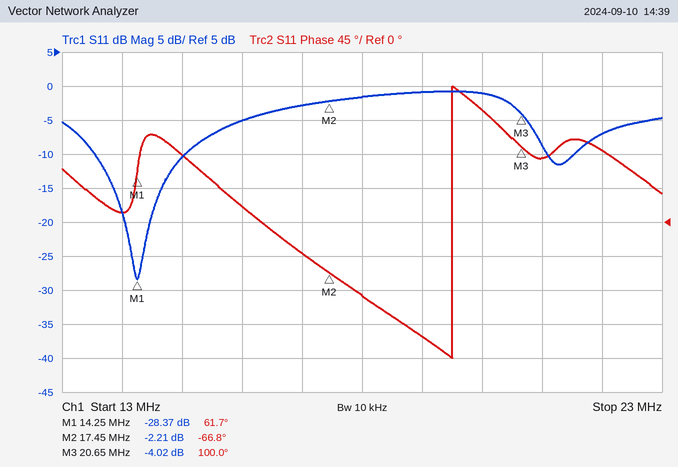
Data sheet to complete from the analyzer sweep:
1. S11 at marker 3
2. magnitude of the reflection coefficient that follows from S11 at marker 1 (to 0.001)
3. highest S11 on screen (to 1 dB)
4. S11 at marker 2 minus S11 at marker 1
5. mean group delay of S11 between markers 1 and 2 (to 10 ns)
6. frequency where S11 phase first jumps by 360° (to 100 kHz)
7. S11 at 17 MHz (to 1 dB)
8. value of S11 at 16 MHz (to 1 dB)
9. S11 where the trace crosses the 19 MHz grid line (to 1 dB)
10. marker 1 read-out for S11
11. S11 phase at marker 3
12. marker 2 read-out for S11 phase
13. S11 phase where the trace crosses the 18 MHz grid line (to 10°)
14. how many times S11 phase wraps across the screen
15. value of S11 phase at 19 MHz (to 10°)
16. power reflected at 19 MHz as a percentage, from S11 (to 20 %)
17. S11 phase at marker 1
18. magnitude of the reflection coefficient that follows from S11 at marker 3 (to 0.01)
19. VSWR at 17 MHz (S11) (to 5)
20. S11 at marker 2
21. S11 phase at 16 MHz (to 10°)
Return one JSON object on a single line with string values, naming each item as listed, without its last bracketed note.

{"S11 at marker 3": "-4.02 dB", "magnitude of the reflection coefficient that follows from S11 at marker 1": "0.038", "highest S11 on screen": "-1 dB", "S11 at marker 2 minus S11 at marker 1": "26.16 dB", "mean group delay of S11 between markers 1 and 2": "110 ns", "frequency where S11 phase first jumps by 360°": "19.5 MHz", "S11 at 17 MHz": "-3 dB", "value of S11 at 16 MHz": "-5 dB", "S11 where the trace crosses the 19 MHz grid line": "-1 dB", "marker 1 read-out for S11": "-28.37 dB", "S11 phase at marker 3": "100.0°", "marker 2 read-out for S11 phase": "-66.8°", "S11 phase where the trace crosses the 18 MHz grid line": "-100°", "how many times S11 phase wraps across the screen": "1", "value of S11 phase at 19 MHz": "-150°", "power reflected at 19 MHz as a percentage, from S11": "80 %", "S11 phase at marker 1": "61.7°", "magnitude of the reflection coefficient that follows from S11 at marker 3": "0.63", "VSWR at 17 MHz (S11)": "5", "S11 at marker 2": "-2.21 dB", "S11 phase at 16 MHz": "20°"}
